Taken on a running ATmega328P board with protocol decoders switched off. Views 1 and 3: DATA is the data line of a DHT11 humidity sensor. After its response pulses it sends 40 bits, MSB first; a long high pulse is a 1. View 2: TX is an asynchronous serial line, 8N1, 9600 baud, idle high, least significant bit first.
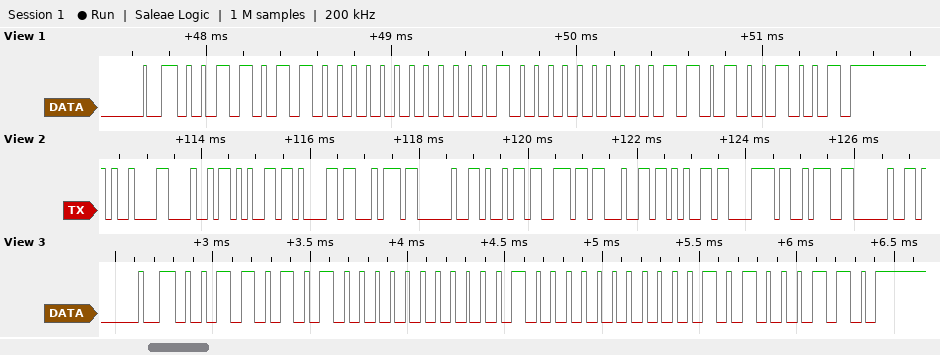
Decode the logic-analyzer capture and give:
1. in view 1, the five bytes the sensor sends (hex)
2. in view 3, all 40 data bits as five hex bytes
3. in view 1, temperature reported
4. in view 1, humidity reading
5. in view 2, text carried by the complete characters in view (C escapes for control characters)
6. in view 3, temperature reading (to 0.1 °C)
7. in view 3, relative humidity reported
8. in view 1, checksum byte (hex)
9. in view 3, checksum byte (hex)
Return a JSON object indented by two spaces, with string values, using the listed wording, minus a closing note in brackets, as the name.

{
  "in view 1, the five bytes the sensor sends": "36 00 10 03 49",
  "in view 3, all 40 data bits as five hex bytes": "35 00 10 01 46",
  "in view 1, temperature reported": "16.3 °C",
  "in view 1, humidity reading": "54 %",
  "in view 2, text carried by the complete characters in view": "\"\\tHeat index: \"",
  "in view 3, temperature reading": "16.1 °C",
  "in view 3, relative humidity reported": "53 %",
  "in view 1, checksum byte": "0x49",
  "in view 3, checksum byte": "0x46"
}
